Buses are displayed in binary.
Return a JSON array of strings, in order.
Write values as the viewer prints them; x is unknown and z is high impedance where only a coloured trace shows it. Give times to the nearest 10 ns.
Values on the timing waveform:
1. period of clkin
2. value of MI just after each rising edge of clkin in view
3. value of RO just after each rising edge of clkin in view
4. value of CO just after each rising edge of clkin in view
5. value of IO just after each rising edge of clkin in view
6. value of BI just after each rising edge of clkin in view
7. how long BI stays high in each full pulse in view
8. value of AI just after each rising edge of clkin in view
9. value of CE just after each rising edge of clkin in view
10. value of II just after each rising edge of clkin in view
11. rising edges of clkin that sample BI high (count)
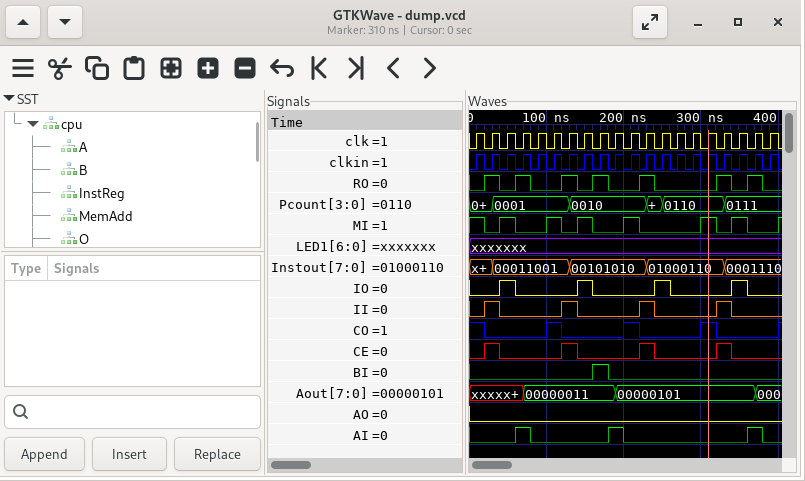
["20 ns", "1 0 1 0 0 1 0 1 0 0 1 0 0 0 0 1 0 1 0 0", "0 1 0 1 0 0 1 0 1 0 0 1 0 0 0 0 1 0 1 0", "1 0 0 0 0 1 0 0 0 0 1 0 0 0 0 1 0 0 0 0", "0 0 1 0 0 0 0 1 0 0 0 0 1 0 0 0 0 1 0 0", "0 0 0 0 0 0 0 0 1 0 0 0 0 0 0 0 0 0 0 0", "20 ns", "0 0 0 1 0 0 0 0 0 1 0 0 0 0 0 0 0 0 1 0", "0 1 0 0 0 0 1 0 0 0 0 1 0 0 0 0 1 0 0 0", "0 1 0 0 0 0 1 0 0 0 0 1 0 0 0 0 1 0 0 0", "1"]
